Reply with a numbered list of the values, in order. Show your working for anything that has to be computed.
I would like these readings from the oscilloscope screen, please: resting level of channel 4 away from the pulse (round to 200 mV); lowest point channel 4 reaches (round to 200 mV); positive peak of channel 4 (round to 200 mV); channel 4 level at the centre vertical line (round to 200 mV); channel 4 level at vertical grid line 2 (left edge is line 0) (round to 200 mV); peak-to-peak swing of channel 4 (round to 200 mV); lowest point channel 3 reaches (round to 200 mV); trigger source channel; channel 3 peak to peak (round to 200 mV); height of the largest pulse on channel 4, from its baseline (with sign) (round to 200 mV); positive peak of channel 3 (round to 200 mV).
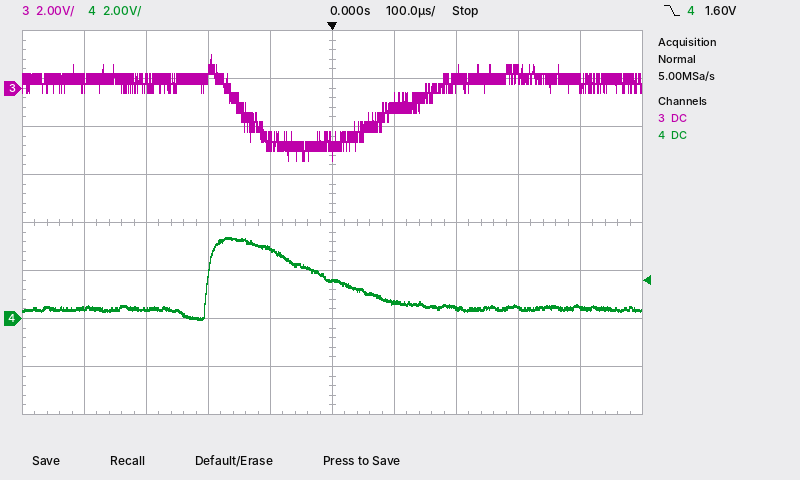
1. 400 mV
2. 0.0 V
3. 3.4 V
4. 1.6 V
5. 400 mV
6. 3.4 V − (0.0 V) = 3.4 V
7. -3.0 V
8. channel 4
9. 1.4 V − (-3.0 V) = 4.4 V
10. 3.4 V − (400 mV) = +3.0 V
11. 1.4 V
